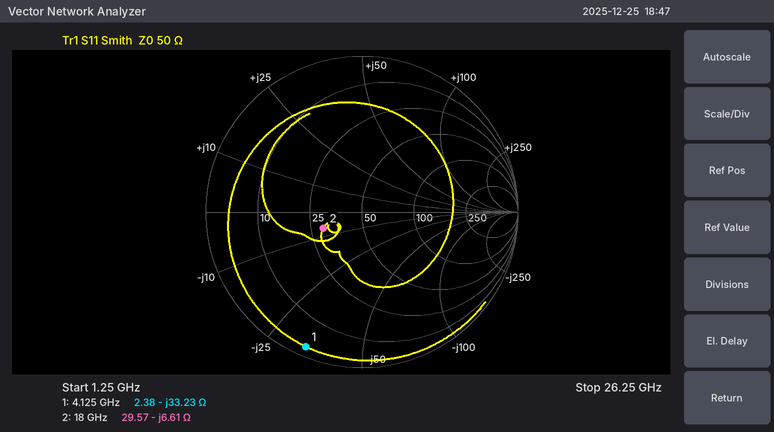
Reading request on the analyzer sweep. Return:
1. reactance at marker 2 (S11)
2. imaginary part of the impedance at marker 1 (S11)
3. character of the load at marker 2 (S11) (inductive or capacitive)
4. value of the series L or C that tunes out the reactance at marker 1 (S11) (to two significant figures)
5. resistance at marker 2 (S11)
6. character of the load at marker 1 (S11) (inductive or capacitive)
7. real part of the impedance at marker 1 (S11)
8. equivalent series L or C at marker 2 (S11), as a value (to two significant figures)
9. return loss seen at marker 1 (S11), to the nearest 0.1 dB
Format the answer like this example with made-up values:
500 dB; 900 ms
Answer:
-6.61 Ω; -33.23 Ω; capacitive; 1.3 nH; 29.57 Ω; capacitive; 2.38 Ω; 1.3 pF; 0.6 dB
